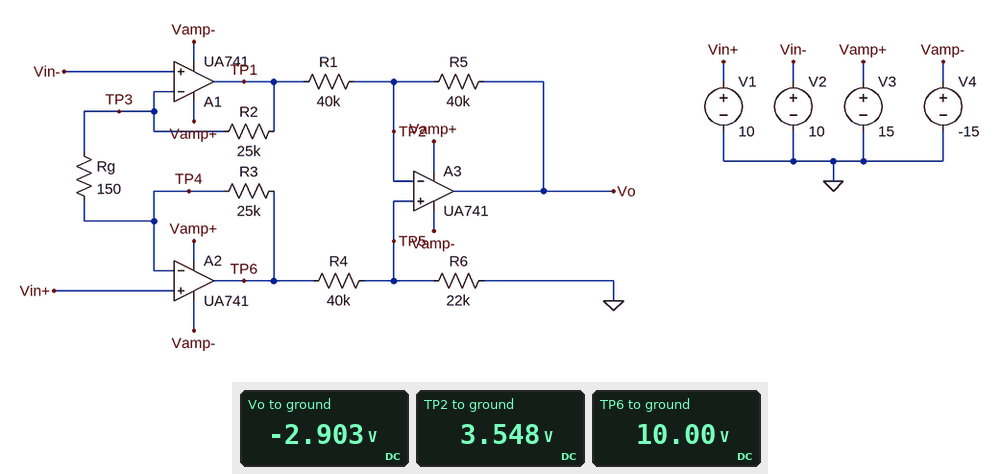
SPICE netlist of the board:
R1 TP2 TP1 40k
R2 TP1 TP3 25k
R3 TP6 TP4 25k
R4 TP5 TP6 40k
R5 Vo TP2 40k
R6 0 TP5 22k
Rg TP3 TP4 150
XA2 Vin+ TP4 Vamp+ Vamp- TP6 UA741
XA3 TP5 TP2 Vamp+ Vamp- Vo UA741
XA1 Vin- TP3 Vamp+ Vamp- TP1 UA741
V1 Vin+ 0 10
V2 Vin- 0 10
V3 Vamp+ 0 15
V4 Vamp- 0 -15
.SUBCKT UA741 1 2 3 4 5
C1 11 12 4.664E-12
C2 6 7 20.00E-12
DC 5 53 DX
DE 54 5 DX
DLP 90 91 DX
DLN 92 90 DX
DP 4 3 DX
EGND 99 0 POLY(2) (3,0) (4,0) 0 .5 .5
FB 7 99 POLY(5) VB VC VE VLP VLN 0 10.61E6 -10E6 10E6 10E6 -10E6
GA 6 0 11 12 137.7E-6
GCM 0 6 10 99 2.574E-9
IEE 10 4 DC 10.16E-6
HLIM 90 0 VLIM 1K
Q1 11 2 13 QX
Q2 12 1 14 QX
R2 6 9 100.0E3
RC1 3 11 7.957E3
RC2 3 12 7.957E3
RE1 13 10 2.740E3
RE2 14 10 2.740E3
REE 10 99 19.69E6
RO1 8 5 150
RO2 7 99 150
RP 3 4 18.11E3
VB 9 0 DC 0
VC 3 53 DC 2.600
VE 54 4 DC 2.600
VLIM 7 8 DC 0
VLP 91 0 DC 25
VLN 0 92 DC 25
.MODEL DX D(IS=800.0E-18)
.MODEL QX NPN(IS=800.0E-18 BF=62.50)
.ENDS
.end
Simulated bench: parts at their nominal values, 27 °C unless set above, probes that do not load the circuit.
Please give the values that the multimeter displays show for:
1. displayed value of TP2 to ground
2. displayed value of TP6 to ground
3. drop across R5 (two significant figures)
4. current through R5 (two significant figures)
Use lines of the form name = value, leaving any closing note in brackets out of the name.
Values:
displayed value of TP2 to ground = 3.548 V
displayed value of TP6 to ground = 10.00 V
drop across R5 = 6.5 V
current through R5 = 160 µA
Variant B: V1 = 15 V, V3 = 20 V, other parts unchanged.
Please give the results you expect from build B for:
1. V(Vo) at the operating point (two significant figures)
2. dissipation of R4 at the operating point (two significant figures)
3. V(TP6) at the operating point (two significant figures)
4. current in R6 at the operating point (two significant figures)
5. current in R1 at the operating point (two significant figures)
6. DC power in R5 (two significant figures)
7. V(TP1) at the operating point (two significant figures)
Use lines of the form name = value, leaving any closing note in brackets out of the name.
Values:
V(Vo) at the operating point = 11 V
dissipation of R4 at the operating point = 3.4 mW
V(TP6) at the operating point = 18 V
current in R6 at the operating point = 290 µA
current in R1 at the operating point = 110 µA
DC power in R5 = 470 µW
V(TP1) at the operating point = 2.0 V
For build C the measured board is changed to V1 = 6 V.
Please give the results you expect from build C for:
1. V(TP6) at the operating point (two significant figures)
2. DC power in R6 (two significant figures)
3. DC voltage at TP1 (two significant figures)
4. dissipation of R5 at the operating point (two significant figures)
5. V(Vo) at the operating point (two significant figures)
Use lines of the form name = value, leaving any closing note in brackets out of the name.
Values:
V(TP6) at the operating point = -960 mV
DC power in R6 = 5.3 µW
DC voltage at TP1 = 13 V
dissipation of R5 at the operating point = 4.2 mW
V(Vo) at the operating point = -13 V
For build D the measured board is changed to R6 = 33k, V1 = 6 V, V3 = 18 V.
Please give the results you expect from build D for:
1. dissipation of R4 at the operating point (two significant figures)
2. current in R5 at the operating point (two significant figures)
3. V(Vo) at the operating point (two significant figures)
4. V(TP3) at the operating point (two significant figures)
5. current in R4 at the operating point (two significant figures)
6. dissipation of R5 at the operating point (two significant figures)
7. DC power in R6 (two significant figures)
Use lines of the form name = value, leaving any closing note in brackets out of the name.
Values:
dissipation of R4 at the operating point = 120 µW
current in R5 at the operating point = 360 µA
V(Vo) at the operating point = -13 V
V(TP3) at the operating point = 6.1 V
current in R4 at the operating point = 54 µA
dissipation of R5 at the operating point = 5.3 mW
DC power in R6 = 96 µW
